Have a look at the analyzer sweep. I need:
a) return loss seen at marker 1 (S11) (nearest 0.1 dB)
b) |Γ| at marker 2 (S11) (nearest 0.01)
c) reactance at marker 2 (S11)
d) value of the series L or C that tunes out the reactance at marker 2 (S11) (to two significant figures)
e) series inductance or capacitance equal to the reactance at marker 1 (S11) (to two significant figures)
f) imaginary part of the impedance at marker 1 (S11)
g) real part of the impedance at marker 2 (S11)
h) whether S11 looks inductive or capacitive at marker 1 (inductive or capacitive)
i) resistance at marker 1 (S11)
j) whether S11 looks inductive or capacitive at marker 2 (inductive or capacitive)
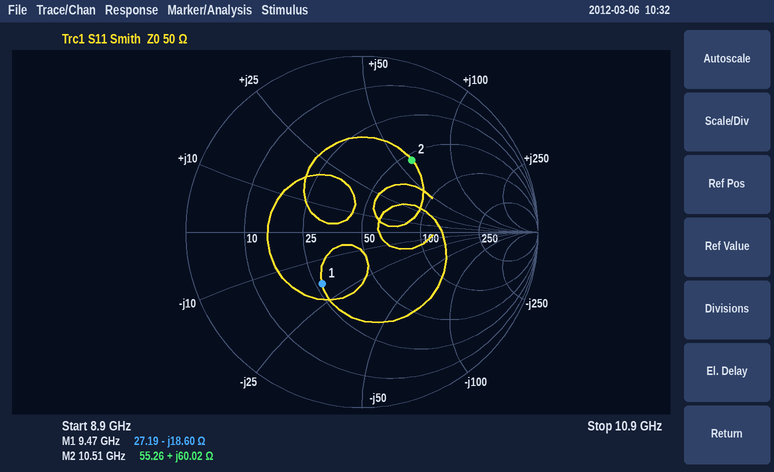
8.6 dB
0.50
+60.02 Ω
250 fF
900 fF
-18.60 Ω
55.26 Ω
capacitive
27.19 Ω
inductive
